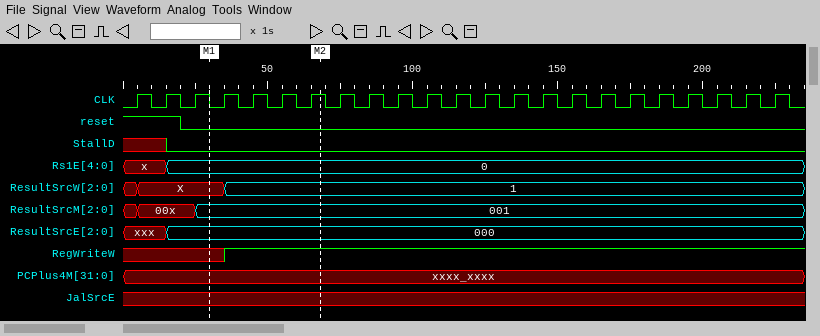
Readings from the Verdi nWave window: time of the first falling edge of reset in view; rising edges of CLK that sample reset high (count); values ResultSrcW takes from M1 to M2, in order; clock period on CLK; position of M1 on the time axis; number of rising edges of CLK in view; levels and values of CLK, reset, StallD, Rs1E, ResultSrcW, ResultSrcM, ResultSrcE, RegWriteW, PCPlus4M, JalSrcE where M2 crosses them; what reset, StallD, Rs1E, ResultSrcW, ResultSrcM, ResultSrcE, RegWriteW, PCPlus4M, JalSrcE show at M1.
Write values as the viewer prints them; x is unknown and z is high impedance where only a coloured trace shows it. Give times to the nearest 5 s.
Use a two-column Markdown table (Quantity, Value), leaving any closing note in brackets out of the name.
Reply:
| Quantity | Value |
|---|---|
| time of the first falling edge of reset in view | 20 s |
| rising edges of CLK that sample reset high | 2 |
| values ResultSrcW takes from M1 to M2, in order | X, 1 |
| clock period on CLK | 10 s |
| position of M1 on the time axis | 30 s |
| number of rising edges of CLK in view | 23 |
| levels and values of CLK, reset, StallD, Rs1E, ResultSrcW, ResultSrcM, ResultSrcE, RegWriteW, PCPlus4M, JalSrcE where M2 crosses them | CLK=1, reset=0, StallD=0, Rs1E=0, ResultSrcW=1, ResultSrcM=001, ResultSrcE=000, RegWriteW=1, PCPlus4M=xxxx_xxxx, JalSrcE=x |
| what reset, StallD, Rs1E, ResultSrcW, ResultSrcM, ResultSrcE, RegWriteW, PCPlus4M, JalSrcE show at M1 | reset=0, StallD=0, Rs1E=0, ResultSrcW=X, ResultSrcM=001, ResultSrcE=000, RegWriteW=x, PCPlus4M=xxxx_xxxx, JalSrcE=x |
